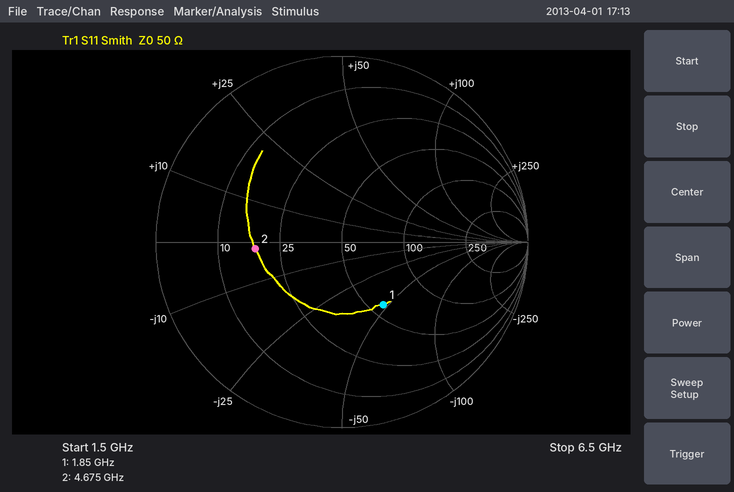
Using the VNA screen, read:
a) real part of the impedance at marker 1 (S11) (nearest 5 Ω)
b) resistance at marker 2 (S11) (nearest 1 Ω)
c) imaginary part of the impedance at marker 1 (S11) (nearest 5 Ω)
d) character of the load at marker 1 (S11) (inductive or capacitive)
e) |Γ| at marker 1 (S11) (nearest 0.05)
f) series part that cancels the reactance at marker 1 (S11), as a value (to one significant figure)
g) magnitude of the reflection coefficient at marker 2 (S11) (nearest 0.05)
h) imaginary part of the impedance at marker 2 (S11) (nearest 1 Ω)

60 Ω
18 Ω
-45 Ω
capacitive
0.40
4 nH
0.45
-2 Ω
